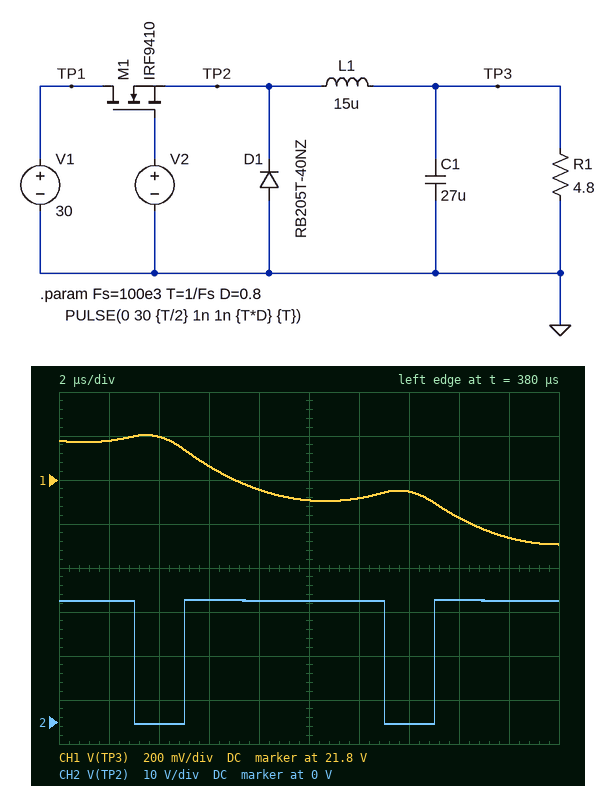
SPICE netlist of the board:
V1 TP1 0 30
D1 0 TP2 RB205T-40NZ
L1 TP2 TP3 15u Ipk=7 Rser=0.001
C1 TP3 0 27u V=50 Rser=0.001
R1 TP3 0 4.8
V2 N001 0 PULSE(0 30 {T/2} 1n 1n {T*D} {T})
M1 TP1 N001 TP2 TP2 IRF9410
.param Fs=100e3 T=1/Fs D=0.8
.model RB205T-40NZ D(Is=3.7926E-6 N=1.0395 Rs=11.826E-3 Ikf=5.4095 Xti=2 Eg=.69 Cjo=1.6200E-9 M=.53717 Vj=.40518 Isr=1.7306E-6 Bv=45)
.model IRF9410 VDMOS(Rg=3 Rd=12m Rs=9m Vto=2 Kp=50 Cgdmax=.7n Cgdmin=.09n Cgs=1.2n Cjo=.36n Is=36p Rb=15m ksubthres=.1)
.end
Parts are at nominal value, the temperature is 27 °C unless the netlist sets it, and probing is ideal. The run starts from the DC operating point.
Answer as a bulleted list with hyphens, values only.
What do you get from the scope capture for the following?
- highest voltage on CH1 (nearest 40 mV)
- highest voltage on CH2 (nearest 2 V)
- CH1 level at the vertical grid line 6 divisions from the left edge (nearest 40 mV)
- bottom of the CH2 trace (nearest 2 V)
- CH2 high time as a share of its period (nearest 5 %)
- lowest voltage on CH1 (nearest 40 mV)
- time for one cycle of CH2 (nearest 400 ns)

- 22.00 V
- 28 V
- 21.72 V
- 0 V
- 80 %
- 21.52 V
- 10.0 µs
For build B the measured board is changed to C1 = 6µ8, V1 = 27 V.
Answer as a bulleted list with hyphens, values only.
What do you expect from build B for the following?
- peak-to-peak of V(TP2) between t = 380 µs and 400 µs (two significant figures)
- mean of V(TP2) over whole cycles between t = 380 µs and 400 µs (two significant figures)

- 27 V
- 21 V
